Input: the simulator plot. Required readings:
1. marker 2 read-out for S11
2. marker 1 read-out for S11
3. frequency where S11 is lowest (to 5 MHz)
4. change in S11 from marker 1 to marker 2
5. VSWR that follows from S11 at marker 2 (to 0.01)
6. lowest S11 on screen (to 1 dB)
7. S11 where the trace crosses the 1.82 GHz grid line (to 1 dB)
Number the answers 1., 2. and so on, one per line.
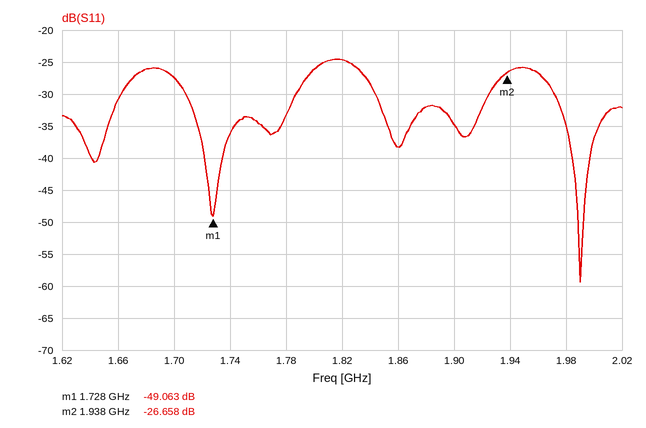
1. -26.658 dB
2. -49.063 dB
3. 1.990 GHz
4. 22.405 dB
5. 1.10
6. -59 dB
7. -25 dB
